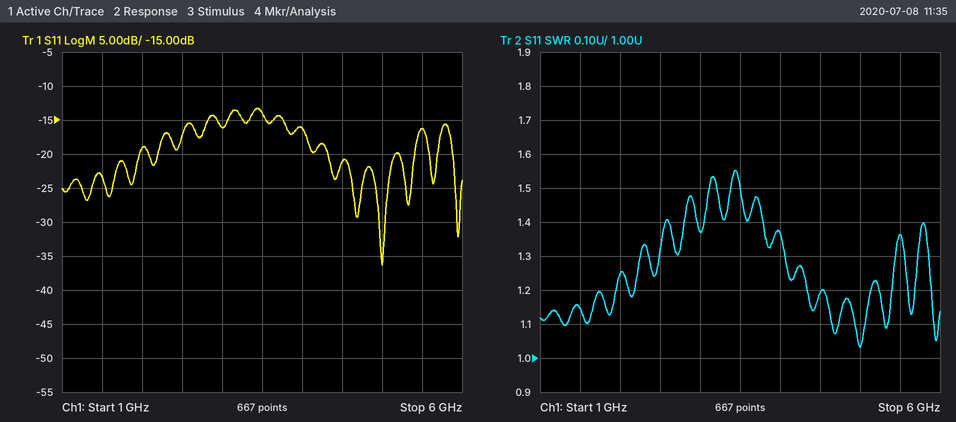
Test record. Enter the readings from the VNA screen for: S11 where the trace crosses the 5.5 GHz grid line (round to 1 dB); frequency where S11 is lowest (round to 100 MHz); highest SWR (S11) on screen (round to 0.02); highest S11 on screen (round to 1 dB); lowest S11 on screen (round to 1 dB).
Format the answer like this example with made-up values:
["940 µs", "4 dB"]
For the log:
["-16 dB", "5.0 GHz", "1.56", "-13 dB", "-36 dB"]
